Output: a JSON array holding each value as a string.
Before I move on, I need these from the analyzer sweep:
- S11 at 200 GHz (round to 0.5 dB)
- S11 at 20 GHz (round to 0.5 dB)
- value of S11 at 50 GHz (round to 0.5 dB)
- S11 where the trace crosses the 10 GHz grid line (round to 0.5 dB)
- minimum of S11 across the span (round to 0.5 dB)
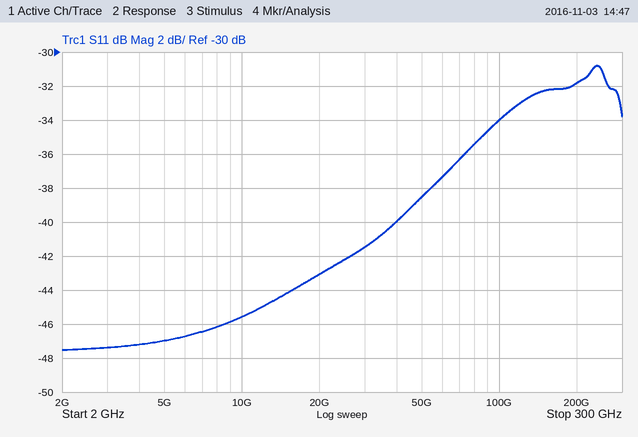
["-32.0 dB", "-43.0 dB", "-38.5 dB", "-45.5 dB", "-47.5 dB"]
